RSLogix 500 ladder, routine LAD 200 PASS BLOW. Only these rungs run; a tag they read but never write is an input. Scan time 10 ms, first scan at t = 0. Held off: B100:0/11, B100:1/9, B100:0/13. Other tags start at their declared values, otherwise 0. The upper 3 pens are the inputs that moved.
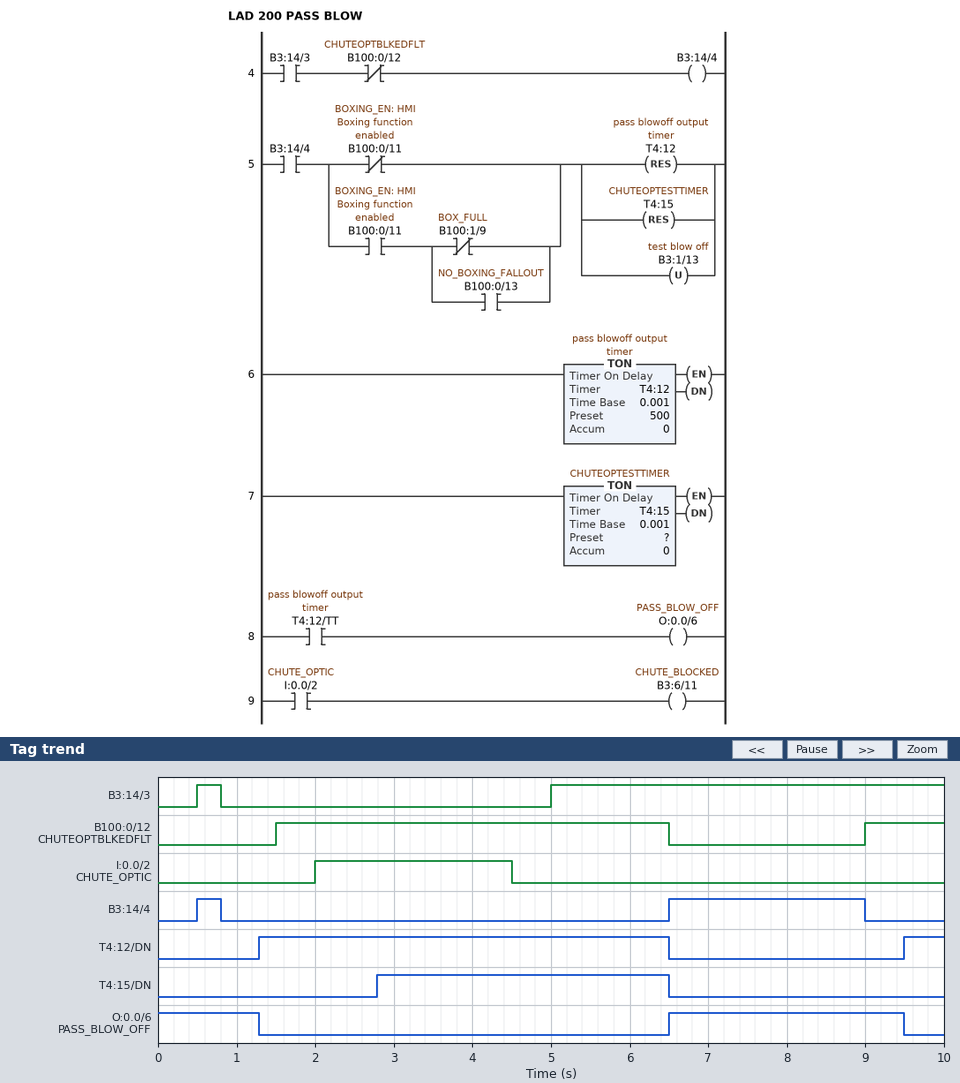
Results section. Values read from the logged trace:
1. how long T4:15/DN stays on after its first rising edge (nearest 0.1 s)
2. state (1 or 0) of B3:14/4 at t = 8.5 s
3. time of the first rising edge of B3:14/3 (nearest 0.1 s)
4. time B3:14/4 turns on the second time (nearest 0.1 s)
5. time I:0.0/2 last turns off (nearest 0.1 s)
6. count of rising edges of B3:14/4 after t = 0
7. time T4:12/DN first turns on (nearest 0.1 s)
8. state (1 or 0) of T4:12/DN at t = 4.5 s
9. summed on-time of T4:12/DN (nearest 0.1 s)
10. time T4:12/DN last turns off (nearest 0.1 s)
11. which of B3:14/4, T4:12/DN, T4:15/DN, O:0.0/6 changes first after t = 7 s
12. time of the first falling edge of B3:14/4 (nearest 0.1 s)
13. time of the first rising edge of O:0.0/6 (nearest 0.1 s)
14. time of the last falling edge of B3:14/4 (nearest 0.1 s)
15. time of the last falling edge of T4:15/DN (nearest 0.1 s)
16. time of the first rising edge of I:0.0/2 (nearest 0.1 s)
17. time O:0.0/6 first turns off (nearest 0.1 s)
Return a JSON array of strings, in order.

["3.7 s", "1", "0.5 s", "6.5 s", "4.5 s", "2", "1.3 s", "1", "5.7 s", "6.5 s", "B3:14/4", "0.8 s", "6.5 s", "9.0 s", "6.5 s", "2.0 s", "1.3 s"]
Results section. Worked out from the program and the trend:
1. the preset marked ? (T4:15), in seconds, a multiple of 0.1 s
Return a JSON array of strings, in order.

["2.0 s"]
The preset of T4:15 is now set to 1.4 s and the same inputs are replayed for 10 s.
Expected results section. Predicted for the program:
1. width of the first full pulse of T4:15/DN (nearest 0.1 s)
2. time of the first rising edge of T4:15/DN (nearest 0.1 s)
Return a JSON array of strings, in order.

["4.3 s", "2.2 s"]
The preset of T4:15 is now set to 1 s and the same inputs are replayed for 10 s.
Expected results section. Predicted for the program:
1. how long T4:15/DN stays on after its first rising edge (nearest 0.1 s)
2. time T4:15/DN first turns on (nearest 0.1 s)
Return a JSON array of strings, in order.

["4.7 s", "1.8 s"]
